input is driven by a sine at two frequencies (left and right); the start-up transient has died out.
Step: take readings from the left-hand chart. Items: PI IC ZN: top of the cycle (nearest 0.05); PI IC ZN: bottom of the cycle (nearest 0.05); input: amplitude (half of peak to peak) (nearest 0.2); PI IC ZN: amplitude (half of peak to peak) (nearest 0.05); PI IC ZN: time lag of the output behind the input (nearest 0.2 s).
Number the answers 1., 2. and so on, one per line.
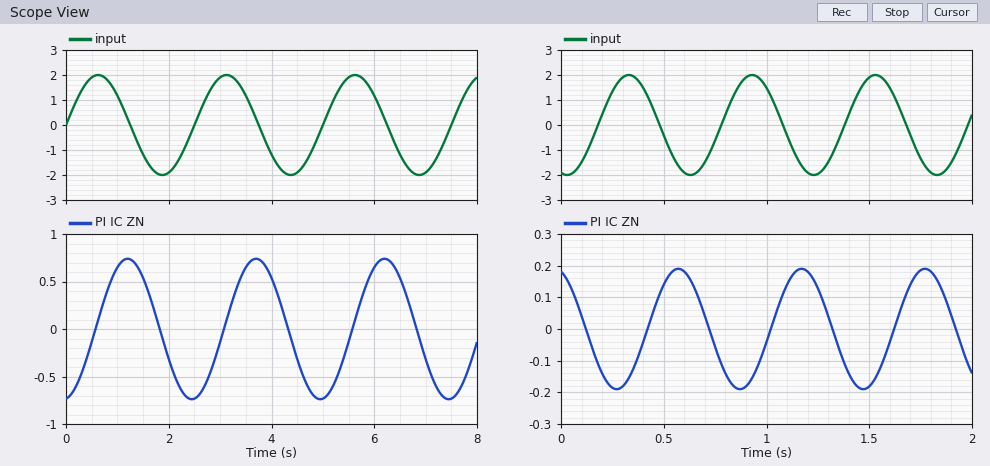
1. 0.75
2. -0.75
3. 2.0
4. 0.75
5. 0.6 s
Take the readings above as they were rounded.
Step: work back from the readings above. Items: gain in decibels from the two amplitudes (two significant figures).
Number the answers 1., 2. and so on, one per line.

1. -8.5 dB
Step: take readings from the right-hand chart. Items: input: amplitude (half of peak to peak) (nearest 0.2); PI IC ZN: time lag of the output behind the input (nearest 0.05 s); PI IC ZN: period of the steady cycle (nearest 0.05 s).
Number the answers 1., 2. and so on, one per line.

1. 2.0
2. 0.25 s
3. 0.60 s
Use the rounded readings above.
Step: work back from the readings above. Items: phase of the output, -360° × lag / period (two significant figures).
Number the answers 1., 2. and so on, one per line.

1. -150°
